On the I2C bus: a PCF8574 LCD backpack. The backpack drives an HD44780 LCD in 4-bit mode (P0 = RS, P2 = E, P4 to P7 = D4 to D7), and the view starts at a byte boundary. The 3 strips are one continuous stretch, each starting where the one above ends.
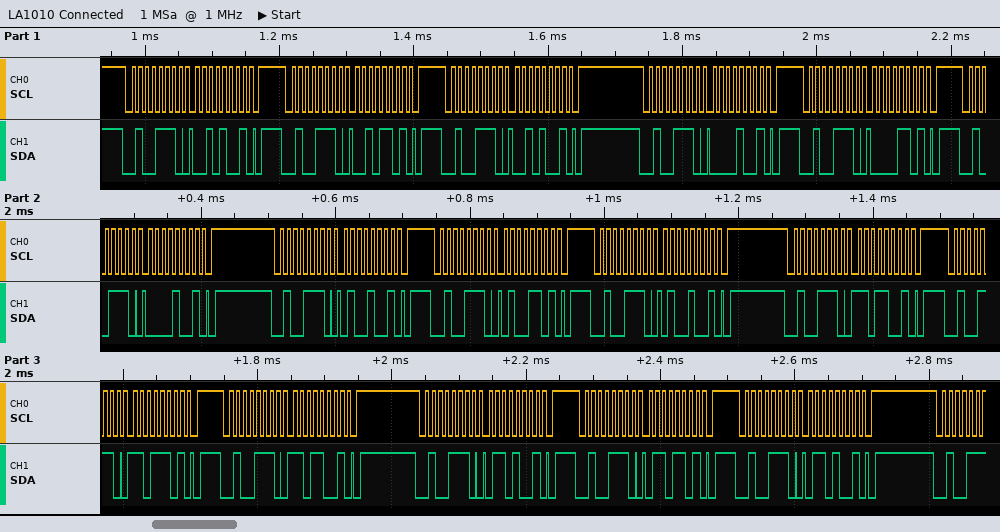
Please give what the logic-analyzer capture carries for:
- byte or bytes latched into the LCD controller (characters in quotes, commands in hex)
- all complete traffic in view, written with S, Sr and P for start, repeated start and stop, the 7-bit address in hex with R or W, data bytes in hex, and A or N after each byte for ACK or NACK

' ' 'M'
S 27W A 29 A P S 27W A 2D A P S 27W A 29 A P S 27W A 09 A P S 27W A 0D A P S 27W A 09 A P S 27W A 49 A P S 27W A 4D A P S 27W A 49 A P S 27W A D9 A P S 27W A DD A P S 27W A D9 A P S 27W A 69 A P S 27W A 6D A P S 27W A 69 A P
